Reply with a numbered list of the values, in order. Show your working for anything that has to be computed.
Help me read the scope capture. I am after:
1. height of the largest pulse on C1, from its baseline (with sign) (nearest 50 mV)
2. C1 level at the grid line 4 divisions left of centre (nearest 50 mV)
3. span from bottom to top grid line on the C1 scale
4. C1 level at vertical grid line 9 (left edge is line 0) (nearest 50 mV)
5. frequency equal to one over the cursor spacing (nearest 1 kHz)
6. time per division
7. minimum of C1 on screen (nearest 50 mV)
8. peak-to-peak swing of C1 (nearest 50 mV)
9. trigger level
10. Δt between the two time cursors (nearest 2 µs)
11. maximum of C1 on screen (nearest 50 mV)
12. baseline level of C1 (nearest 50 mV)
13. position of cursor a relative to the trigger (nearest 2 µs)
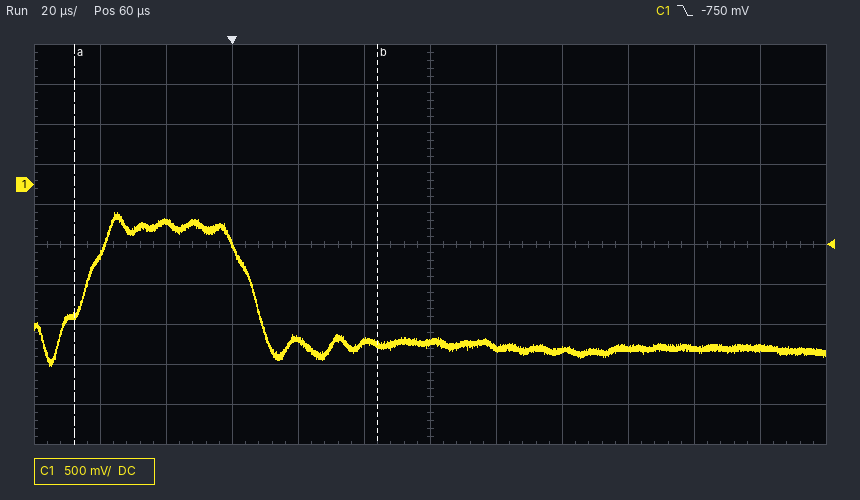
1. -350 mV − (-2.05 V) = +1.70 V
2. -450 mV
3. 5 V
4. -2.05 V
5. 1 / 92 µs ≈ 11 kHz
6. 20 µs
7. -2.25 V
8. -350 mV − (-2.25 V) = 1.90 V
9. -750 mV
10. 92 µs
11. -350 mV
12. -2.05 V
13. -48 µs
